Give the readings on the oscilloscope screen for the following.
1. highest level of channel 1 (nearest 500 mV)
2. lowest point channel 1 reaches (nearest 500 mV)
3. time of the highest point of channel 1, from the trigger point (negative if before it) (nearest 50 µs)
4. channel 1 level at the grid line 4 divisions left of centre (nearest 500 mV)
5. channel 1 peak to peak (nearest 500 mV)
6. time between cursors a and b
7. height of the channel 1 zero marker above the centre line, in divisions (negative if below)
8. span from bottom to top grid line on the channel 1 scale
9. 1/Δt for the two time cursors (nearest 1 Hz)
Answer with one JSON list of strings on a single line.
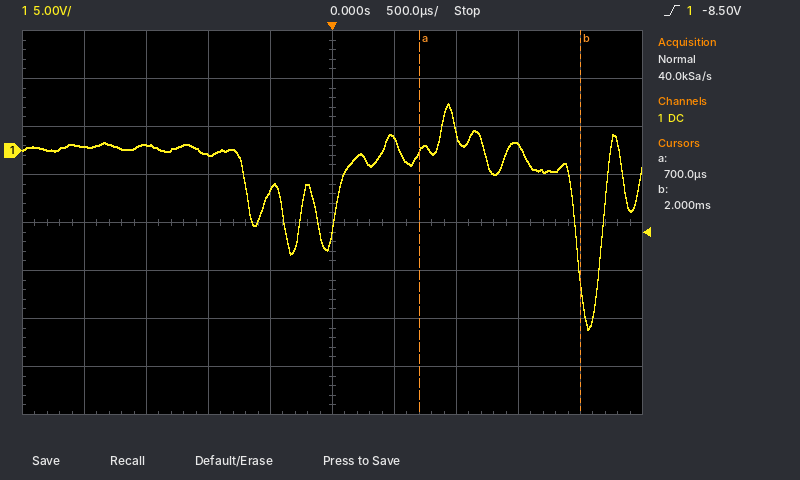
["5.0 V", "-18.5 V", "+950 µs", "500 mV", "23.5 V", "1.30 ms", "+1.5 div", "40 V", "769 Hz"]
